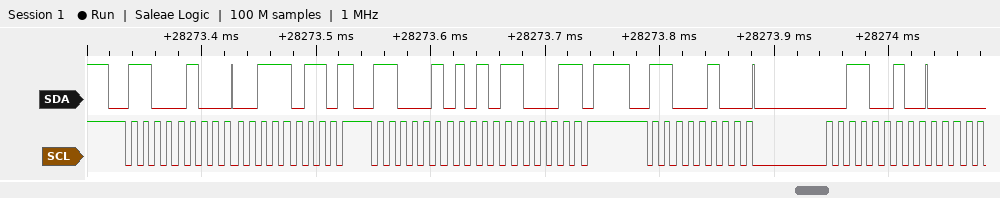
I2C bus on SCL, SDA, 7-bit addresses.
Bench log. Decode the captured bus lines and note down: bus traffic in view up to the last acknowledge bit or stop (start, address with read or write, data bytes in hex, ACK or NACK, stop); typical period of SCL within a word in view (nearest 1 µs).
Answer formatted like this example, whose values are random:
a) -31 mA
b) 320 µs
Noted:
a) start, address 62 write ACK, 3B ACK, repeated start, address 62 read ACK, B1 NACK, stop, start, address 62 write ACK, 32 ACK
b) 10 µs
